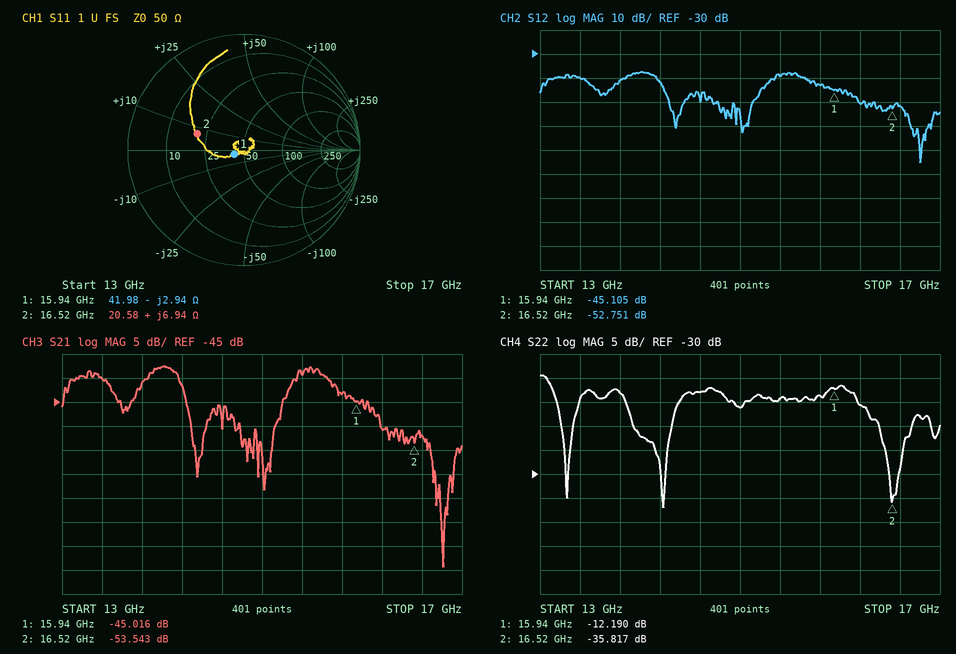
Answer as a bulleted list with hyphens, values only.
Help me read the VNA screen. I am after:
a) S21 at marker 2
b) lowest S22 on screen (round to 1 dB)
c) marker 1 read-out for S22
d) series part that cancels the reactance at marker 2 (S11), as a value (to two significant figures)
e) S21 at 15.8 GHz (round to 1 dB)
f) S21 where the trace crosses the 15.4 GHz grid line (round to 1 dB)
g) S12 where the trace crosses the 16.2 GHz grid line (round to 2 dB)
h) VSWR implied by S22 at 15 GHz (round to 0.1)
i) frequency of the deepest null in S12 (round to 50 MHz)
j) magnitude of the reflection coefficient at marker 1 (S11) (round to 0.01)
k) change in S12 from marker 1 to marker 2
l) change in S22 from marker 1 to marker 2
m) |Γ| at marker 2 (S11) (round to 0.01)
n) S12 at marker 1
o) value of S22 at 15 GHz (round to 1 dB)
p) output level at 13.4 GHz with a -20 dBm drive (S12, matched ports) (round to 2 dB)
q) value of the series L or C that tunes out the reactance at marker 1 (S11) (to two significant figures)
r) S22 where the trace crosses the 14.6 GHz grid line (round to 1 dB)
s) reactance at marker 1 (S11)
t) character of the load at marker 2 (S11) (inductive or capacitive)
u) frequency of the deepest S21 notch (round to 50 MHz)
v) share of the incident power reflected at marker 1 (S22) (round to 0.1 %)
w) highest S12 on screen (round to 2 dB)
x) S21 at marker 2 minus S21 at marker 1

- -53.543 dB
- -37 dB
- -12.190 dB
- 1.4 pF
- -43 dB
- -39 dB
- -50 dB
- 1.4
- 16.80 GHz
- 0.09
- -7.646 dB
- -23.627 dB
- 0.43
- -45.105 dB
- -16 dB
- -60 dBm
- 29 pH
- -13 dB
- -2.94 Ω
- inductive
- 16.80 GHz
- 6.0 %
- -38 dB
- -8.527 dB
